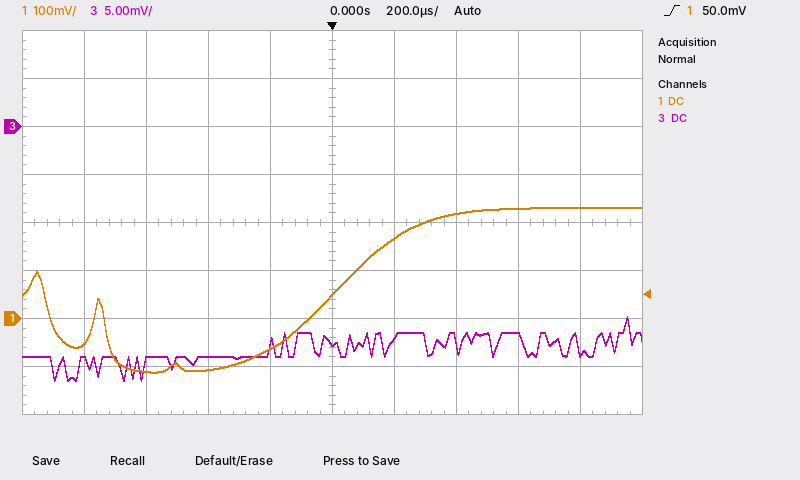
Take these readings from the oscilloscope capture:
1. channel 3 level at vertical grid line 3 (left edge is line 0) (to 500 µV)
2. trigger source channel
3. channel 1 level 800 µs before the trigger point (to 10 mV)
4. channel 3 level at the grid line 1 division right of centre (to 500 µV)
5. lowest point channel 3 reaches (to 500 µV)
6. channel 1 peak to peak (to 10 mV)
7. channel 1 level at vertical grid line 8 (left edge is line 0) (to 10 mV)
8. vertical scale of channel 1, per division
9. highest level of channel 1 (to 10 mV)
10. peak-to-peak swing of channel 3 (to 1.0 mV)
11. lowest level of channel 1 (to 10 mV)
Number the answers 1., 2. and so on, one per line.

1. -24.0 mV
2. channel 1
3. -50 mV
4. -22.0 mV
5. -26.5 mV
6. 340 mV
7. 230 mV
8. 100 mV
9. 230 mV
10. 7.0 mV
11. -110 mV
